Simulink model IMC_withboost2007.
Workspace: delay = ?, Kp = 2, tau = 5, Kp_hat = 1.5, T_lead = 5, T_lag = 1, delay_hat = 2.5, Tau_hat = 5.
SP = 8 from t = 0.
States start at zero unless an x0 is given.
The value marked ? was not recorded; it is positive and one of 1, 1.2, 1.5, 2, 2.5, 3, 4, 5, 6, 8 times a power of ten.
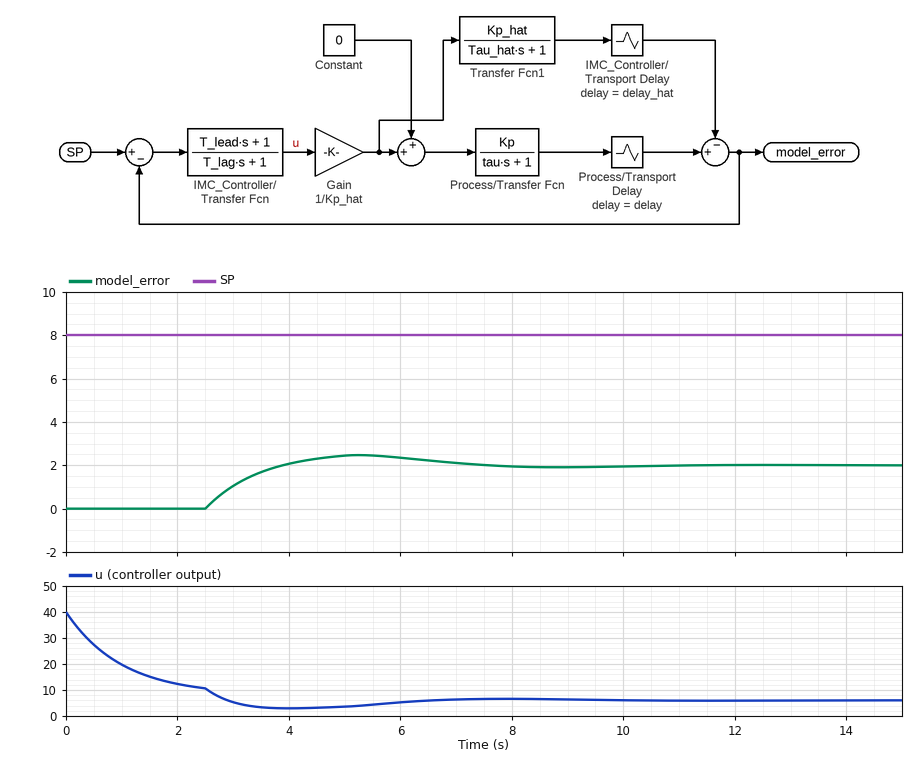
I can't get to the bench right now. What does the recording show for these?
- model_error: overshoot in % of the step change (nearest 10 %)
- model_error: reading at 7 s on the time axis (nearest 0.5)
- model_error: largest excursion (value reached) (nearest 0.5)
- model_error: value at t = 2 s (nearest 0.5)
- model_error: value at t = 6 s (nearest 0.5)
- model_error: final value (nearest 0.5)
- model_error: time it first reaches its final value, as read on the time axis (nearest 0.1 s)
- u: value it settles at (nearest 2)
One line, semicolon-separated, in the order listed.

20 %; 2.0; 2.5; 0.0; 2.5; 2.0; 3.9 s; 6
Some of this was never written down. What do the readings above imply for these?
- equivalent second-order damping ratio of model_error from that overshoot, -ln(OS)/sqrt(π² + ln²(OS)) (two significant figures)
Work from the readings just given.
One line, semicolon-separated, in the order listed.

0.46
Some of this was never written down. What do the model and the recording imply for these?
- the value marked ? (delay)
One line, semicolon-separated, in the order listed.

2.5
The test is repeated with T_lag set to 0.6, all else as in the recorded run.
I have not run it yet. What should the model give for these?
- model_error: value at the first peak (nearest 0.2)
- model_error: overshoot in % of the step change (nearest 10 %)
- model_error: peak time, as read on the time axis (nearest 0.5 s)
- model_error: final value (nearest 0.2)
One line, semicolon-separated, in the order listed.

2.6; 30 %; 5.0 s; 2.0
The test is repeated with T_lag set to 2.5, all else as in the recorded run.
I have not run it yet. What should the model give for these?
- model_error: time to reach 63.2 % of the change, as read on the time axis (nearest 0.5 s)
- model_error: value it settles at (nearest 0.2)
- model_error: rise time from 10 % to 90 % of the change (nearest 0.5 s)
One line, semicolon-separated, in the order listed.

4.0 s; 2.0; 2.5 s
